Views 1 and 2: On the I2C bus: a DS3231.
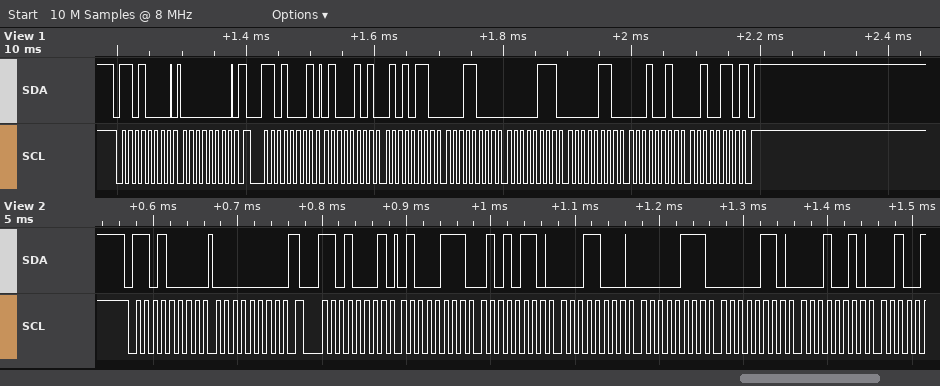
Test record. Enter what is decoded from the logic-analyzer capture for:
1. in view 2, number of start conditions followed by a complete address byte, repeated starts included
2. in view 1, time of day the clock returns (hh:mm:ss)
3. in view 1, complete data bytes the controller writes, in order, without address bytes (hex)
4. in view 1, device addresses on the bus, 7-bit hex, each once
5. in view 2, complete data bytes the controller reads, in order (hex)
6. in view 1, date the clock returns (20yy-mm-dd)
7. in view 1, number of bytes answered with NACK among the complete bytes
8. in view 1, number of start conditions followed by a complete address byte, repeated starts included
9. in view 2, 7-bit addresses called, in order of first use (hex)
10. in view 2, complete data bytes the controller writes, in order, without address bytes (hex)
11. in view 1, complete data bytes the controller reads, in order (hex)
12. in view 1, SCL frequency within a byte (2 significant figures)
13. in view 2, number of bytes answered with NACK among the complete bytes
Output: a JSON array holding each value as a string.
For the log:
["2", "18:56:45", "00", "0x68", "47 56 18 07 06 12", "2026-12-06", "1", "2", "0x68", "00", "45 56 18 07 06 12 26", "100 kHz", "0"]
